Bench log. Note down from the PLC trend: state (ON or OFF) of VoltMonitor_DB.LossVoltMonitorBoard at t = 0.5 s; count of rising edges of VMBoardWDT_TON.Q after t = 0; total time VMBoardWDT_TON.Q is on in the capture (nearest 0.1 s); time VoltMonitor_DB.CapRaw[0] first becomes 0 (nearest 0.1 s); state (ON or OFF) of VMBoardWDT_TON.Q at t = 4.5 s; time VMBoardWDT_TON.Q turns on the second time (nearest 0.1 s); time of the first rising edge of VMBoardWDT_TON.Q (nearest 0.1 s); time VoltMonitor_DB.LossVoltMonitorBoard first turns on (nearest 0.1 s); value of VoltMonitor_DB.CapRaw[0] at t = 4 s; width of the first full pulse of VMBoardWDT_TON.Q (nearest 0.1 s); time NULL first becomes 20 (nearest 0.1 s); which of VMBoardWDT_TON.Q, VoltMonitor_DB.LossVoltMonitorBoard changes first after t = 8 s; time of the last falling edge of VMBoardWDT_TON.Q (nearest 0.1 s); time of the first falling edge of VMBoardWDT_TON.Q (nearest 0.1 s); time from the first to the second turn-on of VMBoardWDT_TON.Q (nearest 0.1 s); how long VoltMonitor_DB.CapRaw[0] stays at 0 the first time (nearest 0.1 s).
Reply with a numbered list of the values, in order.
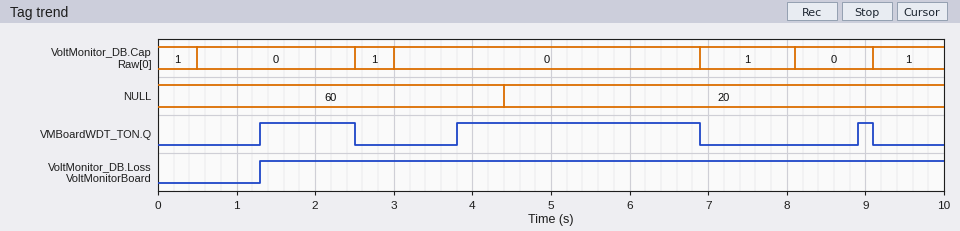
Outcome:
1. OFF
2. 3
3. 4.5 s
4. 0.5 s
5. ON
6. 3.8 s
7. 1.3 s
8. 1.3 s
9. 0
10. 1.2 s
11. 4.4 s
12. VMBoardWDT_TON.Q
13. 9.1 s
14. 2.5 s
15. 2.5 s
16. 2.0 s
